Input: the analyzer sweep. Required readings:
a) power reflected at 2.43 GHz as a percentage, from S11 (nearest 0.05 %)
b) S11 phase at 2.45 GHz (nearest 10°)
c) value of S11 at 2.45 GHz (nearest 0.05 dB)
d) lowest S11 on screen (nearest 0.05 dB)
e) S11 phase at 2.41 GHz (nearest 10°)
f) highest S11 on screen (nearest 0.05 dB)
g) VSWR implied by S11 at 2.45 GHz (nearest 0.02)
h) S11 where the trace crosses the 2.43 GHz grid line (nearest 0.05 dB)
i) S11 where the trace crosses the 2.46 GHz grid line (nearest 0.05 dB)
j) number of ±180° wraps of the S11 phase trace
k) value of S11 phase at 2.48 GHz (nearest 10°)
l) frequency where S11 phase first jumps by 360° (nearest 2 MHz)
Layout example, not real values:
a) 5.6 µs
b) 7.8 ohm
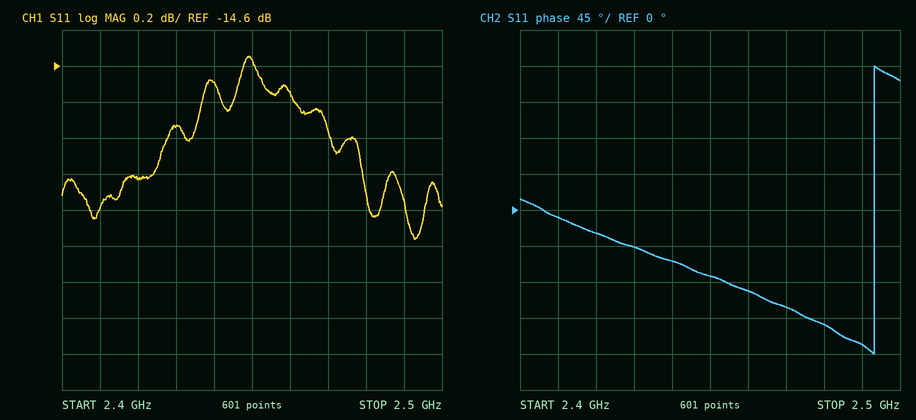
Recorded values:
a) 3.20 %
b) -80°
c) -14.55 dB
d) -15.55 dB
e) -10°
f) -14.55 dB
g) 1.46
h) -14.95 dB
i) -14.75 dB
j) 1
k) -140°
l) 2.494 GHz
